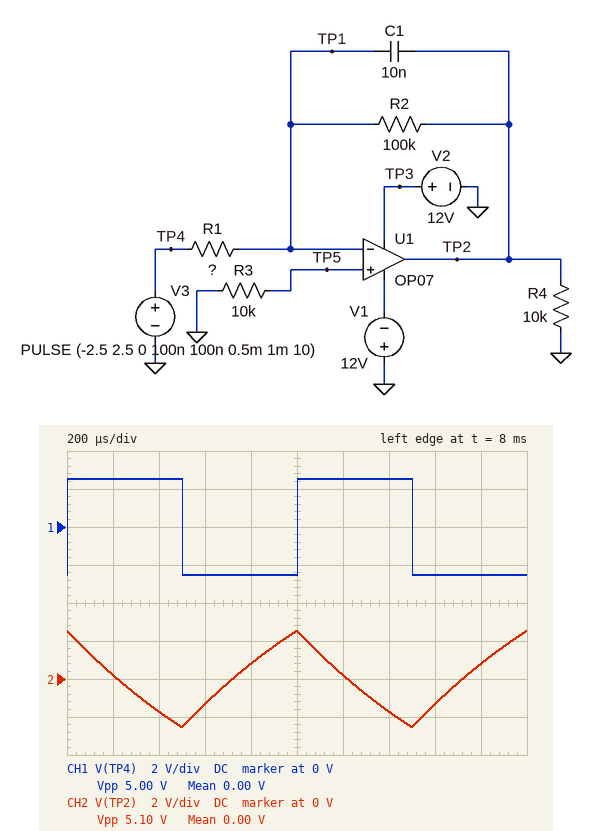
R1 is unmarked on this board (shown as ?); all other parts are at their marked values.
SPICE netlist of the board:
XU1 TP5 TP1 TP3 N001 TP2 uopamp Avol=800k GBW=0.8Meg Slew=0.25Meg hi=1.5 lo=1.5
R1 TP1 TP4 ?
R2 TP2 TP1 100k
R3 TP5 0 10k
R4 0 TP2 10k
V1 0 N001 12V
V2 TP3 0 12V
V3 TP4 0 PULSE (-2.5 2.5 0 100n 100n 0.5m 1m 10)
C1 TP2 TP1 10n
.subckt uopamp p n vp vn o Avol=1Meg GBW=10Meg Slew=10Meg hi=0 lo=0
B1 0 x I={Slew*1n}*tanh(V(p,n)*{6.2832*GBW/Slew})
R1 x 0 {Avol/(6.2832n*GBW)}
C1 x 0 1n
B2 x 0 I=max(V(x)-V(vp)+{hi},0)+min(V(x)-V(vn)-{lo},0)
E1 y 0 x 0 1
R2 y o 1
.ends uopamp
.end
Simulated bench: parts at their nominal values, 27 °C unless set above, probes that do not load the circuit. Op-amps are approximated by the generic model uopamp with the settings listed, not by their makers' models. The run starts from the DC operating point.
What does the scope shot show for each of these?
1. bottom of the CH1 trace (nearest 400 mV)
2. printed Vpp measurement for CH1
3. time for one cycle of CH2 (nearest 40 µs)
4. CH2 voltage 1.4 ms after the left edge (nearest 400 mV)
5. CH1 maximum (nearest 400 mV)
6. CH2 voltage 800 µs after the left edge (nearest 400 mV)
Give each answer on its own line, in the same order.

-2.4 V
5.00 V
1.00 ms
-1.6 V
2.4 V
800 mV
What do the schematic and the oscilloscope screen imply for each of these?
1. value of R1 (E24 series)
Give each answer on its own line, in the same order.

24 kΩ
